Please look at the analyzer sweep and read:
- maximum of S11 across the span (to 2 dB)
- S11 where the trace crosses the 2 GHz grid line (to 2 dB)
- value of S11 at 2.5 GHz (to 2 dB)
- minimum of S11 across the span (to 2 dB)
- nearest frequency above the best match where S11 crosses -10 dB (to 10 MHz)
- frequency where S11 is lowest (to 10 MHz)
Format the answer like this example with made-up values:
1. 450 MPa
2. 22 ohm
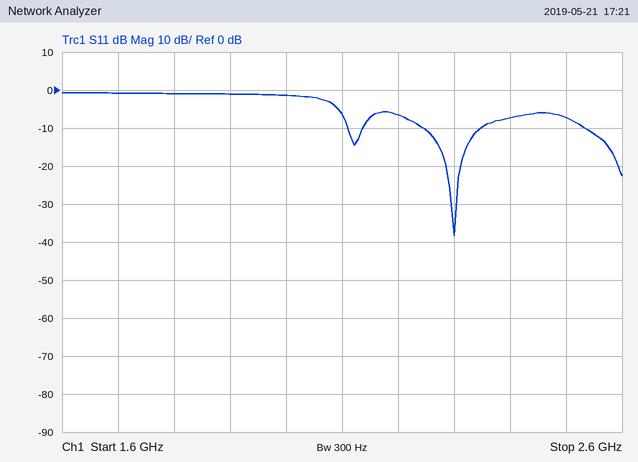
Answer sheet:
1. 0 dB
2. -2 dB
3. -8 dB
4. -38 dB
5. 2.35 GHz
6. 2.30 GHz
